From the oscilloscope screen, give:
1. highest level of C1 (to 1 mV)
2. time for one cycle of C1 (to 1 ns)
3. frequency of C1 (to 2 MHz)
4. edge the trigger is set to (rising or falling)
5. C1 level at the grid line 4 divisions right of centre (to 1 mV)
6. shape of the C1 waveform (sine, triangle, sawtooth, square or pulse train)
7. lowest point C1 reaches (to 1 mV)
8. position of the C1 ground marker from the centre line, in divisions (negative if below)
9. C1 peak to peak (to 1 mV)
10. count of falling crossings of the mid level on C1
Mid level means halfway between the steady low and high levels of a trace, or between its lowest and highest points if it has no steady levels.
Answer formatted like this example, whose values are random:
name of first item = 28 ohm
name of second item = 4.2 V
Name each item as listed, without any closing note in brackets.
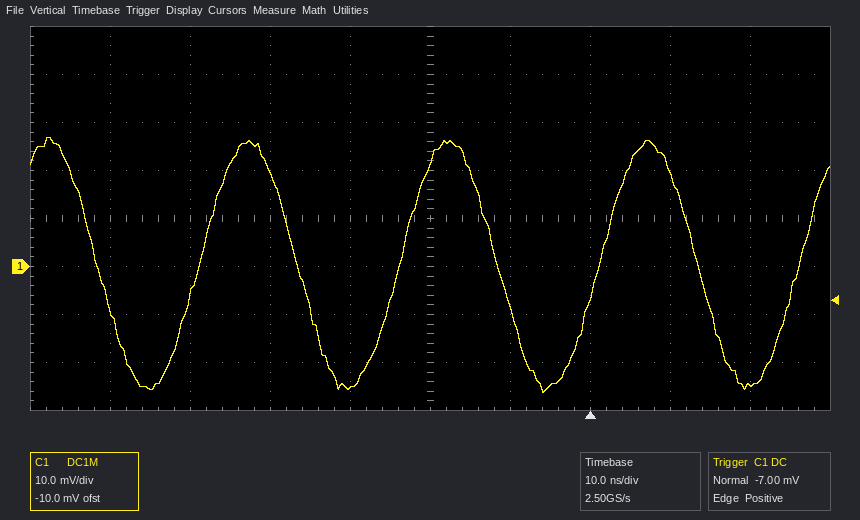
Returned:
highest level of C1 = 27 mV
time for one cycle of C1 = 25 ns
frequency of C1 = 40 MHz
edge the trigger is set to = rising
C1 level at the grid line 4 divisions right of centre = -25 mV
shape of the C1 waveform = sine
lowest point C1 reaches = -26 mV
position of the C1 ground marker from the centre line, in divisions = -1.0 div
C1 peak to peak = 53 mV
count of falling crossings of the mid level on C1 = 4
